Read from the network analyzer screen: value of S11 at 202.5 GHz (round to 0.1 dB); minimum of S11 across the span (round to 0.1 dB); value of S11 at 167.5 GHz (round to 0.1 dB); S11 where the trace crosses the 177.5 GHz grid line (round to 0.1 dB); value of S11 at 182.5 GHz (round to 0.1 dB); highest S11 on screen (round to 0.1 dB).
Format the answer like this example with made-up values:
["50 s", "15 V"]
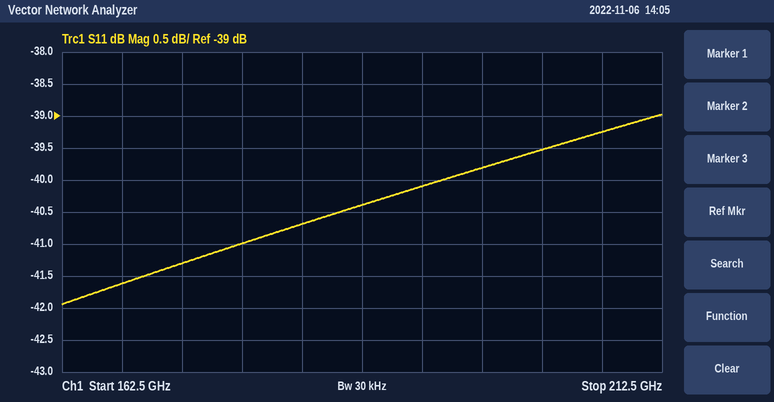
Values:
["-39.5 dB", "-41.9 dB", "-41.6 dB", "-41.0 dB", "-40.7 dB", "-39.0 dB"]
